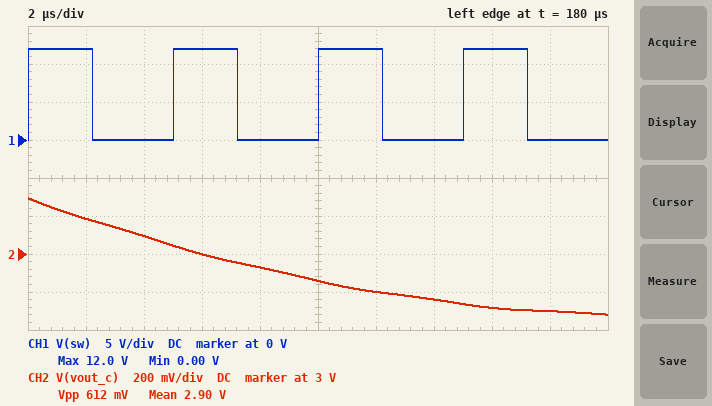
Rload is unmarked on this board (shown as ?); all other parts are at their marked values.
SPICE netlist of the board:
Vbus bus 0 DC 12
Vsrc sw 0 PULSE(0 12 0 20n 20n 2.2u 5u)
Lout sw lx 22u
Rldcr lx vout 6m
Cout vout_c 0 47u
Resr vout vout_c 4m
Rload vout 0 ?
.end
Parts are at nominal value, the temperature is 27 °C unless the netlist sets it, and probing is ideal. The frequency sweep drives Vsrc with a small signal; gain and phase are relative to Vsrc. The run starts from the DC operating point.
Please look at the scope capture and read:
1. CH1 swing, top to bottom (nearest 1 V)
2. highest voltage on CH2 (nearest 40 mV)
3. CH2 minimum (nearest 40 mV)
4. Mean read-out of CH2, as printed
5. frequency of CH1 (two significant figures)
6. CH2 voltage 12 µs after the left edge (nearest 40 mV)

12 V
3.28 V
2.68 V
2.90 V
200 kHz
2.80 V
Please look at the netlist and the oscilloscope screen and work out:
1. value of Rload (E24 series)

3.3 Ω
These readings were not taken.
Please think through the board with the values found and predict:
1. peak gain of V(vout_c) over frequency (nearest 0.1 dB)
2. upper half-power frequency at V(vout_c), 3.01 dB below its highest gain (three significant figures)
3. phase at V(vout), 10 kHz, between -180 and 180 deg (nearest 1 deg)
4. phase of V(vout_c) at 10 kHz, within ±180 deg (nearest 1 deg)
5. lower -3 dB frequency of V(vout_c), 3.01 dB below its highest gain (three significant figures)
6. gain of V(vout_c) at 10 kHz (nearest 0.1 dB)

13.1 dB
5.41 kHz
-171 deg
-172 deg
4.30 kHz
-9.9 dB
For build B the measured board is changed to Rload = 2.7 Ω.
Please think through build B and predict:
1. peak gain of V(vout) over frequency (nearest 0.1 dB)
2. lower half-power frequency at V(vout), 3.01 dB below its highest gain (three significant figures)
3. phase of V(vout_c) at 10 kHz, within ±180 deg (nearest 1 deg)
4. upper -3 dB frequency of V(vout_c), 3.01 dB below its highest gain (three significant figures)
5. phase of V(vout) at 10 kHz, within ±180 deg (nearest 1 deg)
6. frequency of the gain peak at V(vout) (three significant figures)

11.5 dB
4.14 kHz
-170 deg
5.49 kHz
-169 deg
4.86 kHz
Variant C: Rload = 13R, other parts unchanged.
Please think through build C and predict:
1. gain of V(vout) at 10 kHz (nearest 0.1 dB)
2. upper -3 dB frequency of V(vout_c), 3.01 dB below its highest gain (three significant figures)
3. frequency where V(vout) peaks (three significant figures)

-9.8 dB
5.11 kHz
4.94 kHz
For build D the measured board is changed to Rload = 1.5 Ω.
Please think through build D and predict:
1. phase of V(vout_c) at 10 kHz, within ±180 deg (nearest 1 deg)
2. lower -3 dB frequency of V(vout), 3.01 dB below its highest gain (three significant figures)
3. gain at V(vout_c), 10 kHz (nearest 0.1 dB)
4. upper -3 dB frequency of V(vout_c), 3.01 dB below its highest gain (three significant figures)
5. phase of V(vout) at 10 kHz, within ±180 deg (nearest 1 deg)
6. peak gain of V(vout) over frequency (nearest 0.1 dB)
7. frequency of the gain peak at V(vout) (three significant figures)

-163 deg
3.26 kHz
-10.2 dB
5.75 kHz
-162 deg
6.8 dB
4.67 kHz
